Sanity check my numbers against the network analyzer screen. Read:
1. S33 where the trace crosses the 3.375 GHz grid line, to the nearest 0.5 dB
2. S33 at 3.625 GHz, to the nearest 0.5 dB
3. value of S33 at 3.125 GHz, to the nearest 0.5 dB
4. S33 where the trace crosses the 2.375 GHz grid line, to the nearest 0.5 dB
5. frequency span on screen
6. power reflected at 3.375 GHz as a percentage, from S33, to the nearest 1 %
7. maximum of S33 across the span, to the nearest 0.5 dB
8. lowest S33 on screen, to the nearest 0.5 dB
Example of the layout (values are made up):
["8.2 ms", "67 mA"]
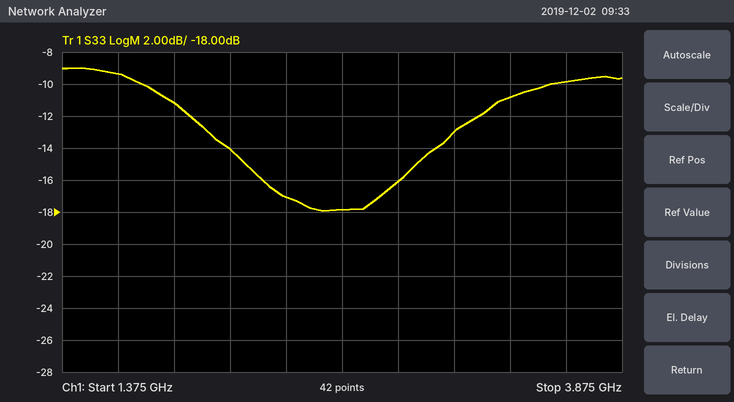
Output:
["-11.0 dB", "-10.0 dB", "-13.0 dB", "-17.0 dB", "2.5 GHz", "8 %", "-9.0 dB", "-18.0 dB"]
